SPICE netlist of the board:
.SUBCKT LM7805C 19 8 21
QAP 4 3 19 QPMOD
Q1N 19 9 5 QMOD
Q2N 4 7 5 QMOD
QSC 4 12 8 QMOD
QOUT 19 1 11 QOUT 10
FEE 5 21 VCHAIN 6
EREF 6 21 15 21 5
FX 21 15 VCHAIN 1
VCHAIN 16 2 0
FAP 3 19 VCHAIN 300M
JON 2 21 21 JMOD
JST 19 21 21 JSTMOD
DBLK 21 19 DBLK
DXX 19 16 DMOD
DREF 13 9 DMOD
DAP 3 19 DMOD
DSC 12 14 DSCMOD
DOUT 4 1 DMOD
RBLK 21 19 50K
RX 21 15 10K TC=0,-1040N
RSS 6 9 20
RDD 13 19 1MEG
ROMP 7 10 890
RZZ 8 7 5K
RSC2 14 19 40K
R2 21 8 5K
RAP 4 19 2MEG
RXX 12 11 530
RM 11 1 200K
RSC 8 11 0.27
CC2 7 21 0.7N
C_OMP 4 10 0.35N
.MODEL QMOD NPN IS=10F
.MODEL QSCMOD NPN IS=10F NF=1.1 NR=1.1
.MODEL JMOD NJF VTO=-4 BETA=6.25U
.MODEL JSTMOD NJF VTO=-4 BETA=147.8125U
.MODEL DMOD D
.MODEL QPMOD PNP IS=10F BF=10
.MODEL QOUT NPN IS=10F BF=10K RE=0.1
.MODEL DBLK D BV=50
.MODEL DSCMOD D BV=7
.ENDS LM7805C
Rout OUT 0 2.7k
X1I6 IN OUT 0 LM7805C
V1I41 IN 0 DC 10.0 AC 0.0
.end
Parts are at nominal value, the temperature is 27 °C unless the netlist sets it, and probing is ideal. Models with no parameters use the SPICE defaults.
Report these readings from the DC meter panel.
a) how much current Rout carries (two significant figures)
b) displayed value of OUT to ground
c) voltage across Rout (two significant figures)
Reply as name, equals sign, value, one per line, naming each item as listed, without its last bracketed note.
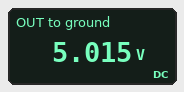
how much current Rout carries = 1.9 mA
displayed value of OUT to ground = 5.015 V
voltage across Rout = 5.0 V
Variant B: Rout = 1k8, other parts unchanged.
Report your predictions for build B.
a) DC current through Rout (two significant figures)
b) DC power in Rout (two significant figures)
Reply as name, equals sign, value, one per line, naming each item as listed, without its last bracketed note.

DC current through Rout = 2.8 mA
DC power in Rout = 14 mW
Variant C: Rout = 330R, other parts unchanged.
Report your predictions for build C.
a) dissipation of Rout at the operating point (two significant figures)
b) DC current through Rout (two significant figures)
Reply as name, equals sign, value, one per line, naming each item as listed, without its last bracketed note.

dissipation of Rout at the operating point = 76 mW
DC current through Rout = 15 mA
